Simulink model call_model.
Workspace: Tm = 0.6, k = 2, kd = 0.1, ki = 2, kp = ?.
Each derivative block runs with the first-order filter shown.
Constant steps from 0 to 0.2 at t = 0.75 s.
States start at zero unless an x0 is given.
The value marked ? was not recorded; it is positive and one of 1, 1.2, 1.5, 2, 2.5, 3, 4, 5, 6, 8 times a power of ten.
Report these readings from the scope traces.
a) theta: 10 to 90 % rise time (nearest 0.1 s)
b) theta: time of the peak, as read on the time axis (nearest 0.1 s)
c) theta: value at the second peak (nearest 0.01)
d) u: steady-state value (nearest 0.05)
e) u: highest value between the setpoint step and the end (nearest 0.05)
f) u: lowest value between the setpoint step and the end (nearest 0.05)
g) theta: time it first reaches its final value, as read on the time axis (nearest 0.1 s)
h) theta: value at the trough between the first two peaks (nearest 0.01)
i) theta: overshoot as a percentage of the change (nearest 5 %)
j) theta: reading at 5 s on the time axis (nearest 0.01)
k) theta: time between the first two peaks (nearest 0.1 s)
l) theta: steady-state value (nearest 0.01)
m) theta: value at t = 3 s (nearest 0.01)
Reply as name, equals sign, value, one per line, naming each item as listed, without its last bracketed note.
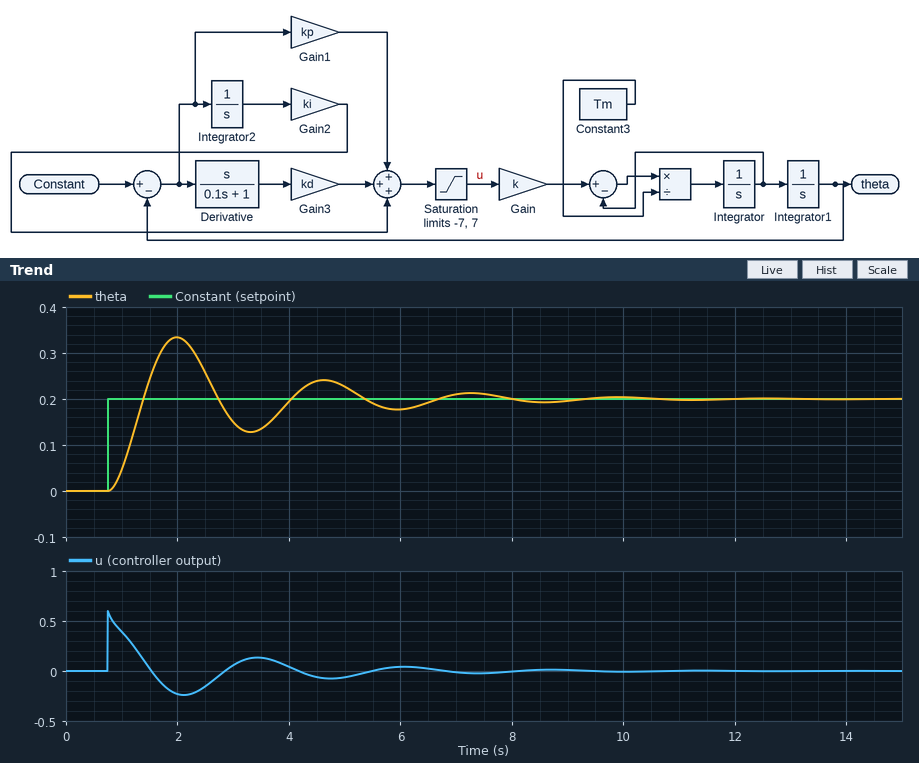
theta: 10 to 90 % rise time = 0.4 s
theta: time of the peak, as read on the time axis = 2.0 s
theta: value at the second peak = 0.24
u: steady-state value = 0.00
u: highest value between the setpoint step and the end = 0.60
u: lowest value between the setpoint step and the end = -0.25
theta: time it first reaches its final value, as read on the time axis = 1.4 s
theta: value at the trough between the first two peaks = 0.13
theta: overshoot as a percentage of the change = 65 %
theta: reading at 5 s on the time axis = 0.23
theta: time between the first two peaks = 2.6 s
theta: steady-state value = 0.20
theta: value at t = 3 s = 0.15
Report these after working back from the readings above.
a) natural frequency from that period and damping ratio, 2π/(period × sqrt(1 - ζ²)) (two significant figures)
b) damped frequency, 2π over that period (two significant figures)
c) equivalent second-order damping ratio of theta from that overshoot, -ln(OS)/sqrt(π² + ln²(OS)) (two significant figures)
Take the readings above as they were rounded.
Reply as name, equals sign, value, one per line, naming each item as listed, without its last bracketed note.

natural frequency from that period and damping ratio, 2π/(period × sqrt(1 - ζ²)) = 2.4 rad/s
damped frequency, 2π over that period = 2.4 rad/s
equivalent second-order damping ratio of theta from that overshoot, -ln(OS)/sqrt(π² + ln²(OS)) = 0.14
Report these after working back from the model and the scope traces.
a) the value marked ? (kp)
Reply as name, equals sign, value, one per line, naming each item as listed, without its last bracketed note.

the value marked ? = 2
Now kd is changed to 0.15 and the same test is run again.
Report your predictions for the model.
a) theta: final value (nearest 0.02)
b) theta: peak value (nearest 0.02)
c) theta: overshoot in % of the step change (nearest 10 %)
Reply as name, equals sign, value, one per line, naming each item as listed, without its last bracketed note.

theta: final value = 0.20
theta: peak value = 0.32
theta: overshoot in % of the step change = 60 %
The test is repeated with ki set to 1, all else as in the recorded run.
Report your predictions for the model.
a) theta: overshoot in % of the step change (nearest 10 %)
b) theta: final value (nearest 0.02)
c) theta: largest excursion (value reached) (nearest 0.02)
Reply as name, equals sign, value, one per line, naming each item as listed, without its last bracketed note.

theta: overshoot in % of the step change = 50 %
theta: final value = 0.20
theta: largest excursion (value reached) = 0.30
